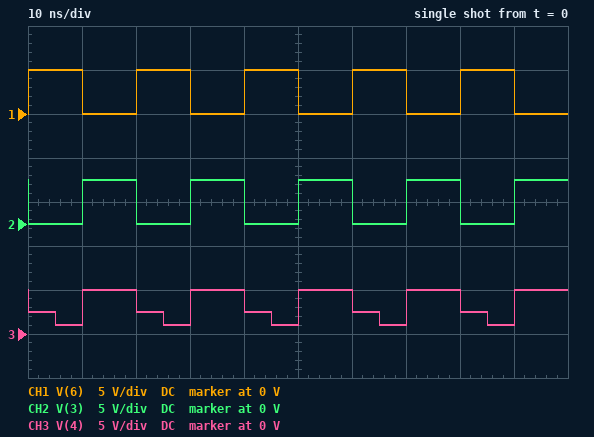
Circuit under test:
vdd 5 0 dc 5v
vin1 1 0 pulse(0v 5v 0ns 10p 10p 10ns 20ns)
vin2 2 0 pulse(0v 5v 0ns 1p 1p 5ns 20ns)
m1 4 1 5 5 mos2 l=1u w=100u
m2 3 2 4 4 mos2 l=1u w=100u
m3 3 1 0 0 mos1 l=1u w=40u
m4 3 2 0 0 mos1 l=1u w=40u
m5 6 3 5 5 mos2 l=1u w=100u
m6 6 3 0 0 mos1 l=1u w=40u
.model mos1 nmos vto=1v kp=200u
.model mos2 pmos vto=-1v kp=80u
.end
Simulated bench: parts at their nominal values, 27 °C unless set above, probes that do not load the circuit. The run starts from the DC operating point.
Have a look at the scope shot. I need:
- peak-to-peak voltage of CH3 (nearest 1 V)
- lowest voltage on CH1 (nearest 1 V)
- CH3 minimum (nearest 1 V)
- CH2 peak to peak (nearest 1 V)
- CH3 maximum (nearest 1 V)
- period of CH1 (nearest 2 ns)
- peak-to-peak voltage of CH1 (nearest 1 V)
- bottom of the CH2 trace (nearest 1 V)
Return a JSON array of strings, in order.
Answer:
["4 V", "0 V", "1 V", "5 V", "5 V", "20 ns", "5 V", "0 V"]
